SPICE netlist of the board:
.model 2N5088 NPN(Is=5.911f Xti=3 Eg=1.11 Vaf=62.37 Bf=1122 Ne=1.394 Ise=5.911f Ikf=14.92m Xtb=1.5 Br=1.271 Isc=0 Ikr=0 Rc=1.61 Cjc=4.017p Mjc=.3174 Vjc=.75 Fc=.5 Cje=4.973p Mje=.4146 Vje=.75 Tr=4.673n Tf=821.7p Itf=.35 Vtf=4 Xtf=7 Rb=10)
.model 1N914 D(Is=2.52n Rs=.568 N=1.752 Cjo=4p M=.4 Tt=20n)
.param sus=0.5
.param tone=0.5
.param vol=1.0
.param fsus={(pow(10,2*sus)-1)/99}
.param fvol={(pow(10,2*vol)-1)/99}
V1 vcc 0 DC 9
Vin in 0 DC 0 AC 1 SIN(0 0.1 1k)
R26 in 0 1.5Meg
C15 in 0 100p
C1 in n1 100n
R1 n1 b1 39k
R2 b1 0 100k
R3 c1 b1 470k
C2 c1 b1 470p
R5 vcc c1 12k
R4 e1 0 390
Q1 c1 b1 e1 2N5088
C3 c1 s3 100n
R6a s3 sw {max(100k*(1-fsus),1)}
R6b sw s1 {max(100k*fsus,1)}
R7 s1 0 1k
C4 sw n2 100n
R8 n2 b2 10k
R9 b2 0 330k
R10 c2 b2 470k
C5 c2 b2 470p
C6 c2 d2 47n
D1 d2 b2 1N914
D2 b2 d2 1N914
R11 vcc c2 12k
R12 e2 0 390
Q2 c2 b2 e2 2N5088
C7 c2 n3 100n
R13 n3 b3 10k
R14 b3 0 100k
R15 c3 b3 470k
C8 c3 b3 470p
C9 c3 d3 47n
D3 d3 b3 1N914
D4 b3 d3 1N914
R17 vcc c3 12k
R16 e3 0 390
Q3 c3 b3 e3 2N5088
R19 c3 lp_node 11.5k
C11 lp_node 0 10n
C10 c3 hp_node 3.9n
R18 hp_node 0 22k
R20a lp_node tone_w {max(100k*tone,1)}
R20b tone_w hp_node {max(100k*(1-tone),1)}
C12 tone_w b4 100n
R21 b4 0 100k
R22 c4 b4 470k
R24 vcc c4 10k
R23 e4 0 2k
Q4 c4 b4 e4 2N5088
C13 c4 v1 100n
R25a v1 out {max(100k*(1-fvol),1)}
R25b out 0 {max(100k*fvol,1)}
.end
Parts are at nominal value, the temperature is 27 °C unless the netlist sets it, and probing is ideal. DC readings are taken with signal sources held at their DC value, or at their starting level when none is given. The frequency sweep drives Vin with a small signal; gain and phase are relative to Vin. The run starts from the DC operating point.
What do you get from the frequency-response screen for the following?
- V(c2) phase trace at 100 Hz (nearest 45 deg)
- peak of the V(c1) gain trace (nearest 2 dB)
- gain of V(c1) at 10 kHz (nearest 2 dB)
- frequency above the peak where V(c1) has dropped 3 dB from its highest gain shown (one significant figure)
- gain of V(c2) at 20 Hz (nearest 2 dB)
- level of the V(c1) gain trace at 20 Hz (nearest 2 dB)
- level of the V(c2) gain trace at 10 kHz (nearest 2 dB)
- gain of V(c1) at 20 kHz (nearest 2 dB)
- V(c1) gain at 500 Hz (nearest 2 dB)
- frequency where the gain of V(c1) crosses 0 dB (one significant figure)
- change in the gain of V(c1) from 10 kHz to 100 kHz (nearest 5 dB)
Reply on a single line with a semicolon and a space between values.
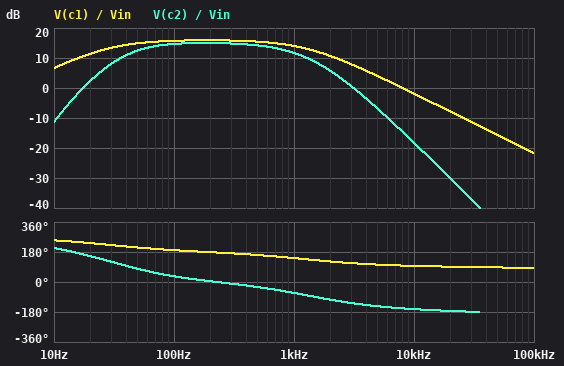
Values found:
45 deg; 16 dB; -2 dB; 1 kHz; 2 dB; 12 dB; -18 dB; -8 dB; 16 dB; 8 kHz; -20 dB
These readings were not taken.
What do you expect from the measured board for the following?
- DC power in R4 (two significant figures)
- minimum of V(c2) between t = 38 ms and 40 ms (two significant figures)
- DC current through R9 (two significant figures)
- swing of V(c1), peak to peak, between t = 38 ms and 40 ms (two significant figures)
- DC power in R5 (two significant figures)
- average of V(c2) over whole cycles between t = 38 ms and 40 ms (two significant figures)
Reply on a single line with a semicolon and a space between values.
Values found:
48 µW; 2.3 V; 2.6 µA; 1.0 V; 1.5 mW; 2.5 V
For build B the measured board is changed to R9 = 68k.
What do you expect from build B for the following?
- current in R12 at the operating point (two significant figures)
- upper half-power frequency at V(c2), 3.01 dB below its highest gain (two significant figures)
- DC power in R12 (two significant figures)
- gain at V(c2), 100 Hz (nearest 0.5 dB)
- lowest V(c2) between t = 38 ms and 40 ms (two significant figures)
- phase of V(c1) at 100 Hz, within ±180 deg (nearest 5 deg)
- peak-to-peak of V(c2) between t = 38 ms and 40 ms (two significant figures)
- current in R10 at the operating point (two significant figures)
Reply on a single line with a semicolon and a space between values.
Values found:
240 µA; 1.0 kHz; 23 µW; 13.0 dB; 5.7 V; -170 deg; 460 mV; 11 µA
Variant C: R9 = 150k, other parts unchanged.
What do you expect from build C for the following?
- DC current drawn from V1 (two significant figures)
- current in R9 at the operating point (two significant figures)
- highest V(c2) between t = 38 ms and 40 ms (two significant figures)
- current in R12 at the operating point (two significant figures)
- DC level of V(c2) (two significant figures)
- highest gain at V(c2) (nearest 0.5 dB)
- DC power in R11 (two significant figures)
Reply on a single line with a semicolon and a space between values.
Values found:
1.4 mA; 5.4 µA; 4.0 V; 430 µA; 3.7 V; 14.5 dB; 2.3 mW
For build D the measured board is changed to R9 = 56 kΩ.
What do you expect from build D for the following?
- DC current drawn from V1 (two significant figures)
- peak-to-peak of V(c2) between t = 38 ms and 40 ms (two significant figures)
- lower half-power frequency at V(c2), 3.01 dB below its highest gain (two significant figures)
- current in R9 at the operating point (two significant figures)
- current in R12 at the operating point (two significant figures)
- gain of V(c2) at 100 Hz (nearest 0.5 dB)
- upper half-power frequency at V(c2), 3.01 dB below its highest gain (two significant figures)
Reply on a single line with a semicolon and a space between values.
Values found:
1.2 mA; 440 mV; 47 Hz; 12 µA; 180 µA; 12.5 dB; 1.0 kHz
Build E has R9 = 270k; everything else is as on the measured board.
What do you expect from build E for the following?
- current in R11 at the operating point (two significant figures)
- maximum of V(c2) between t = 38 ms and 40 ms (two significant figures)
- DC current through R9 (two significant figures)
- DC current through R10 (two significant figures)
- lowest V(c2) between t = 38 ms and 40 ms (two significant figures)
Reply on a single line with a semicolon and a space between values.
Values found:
520 µA; 3.0 V; 3.2 µA; 4.0 µA; 2.5 V
